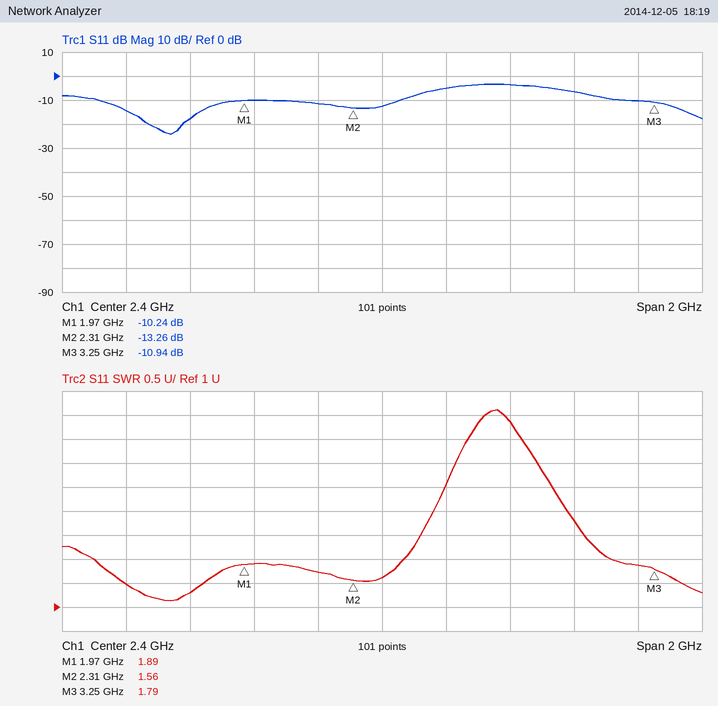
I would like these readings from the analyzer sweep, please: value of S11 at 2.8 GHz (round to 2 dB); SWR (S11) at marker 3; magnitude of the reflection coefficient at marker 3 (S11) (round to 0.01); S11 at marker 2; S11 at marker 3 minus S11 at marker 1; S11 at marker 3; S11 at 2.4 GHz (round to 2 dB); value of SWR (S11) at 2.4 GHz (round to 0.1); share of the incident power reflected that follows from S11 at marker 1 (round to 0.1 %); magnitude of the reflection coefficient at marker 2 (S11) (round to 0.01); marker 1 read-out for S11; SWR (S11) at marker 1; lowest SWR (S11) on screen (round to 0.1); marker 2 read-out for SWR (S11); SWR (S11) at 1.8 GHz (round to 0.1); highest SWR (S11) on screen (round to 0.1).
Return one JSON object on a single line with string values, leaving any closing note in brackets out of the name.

{"value of S11 at 2.8 GHz": "-4 dB", "SWR (S11) at marker 3": "1.79", "magnitude of the reflection coefficient at marker 3 (S11)": "0.28", "S11 at marker 2": "-13.26 dB", "S11 at marker 3 minus S11 at marker 1": "-0.70 dB", "S11 at marker 3": "-10.94 dB", "S11 at 2.4 GHz": "-12 dB", "value of SWR (S11) at 2.4 GHz": "1.6", "share of the incident power reflected that follows from S11 at marker 1": "9.5 %", "magnitude of the reflection coefficient at marker 2 (S11)": "0.22", "marker 1 read-out for S11": "-10.24 dB", "SWR (S11) at marker 1": "1.89", "lowest SWR (S11) on screen": "1.1", "marker 2 read-out for SWR": "1.56", "SWR (S11) at 1.8 GHz": "1.3", "highest SWR (S11) on screen": "5.1"}
